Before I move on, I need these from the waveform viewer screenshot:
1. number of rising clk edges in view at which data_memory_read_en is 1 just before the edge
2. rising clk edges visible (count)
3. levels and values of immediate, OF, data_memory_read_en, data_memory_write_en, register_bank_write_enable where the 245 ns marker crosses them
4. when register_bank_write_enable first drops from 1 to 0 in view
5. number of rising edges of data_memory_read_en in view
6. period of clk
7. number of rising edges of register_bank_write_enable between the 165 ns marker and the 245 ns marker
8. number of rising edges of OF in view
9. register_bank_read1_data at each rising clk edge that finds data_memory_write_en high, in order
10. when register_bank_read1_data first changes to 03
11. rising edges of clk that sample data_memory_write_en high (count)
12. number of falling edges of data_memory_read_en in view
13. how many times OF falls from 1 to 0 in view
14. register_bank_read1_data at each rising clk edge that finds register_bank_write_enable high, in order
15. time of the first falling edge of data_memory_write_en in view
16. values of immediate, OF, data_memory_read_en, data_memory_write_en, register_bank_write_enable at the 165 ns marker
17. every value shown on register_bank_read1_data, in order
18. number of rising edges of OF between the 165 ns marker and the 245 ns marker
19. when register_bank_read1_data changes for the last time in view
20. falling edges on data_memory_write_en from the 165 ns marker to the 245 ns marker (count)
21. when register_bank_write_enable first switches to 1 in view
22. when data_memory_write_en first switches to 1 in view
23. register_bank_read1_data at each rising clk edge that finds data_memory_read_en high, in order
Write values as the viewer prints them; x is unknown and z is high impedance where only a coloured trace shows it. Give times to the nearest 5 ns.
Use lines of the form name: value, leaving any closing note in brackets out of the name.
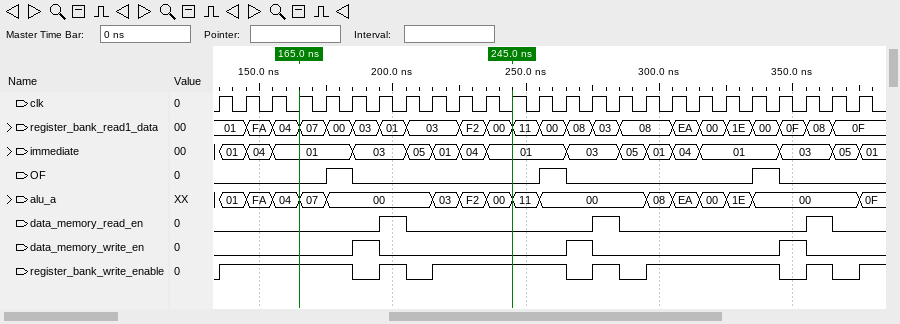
number of rising clk edges in view at which data_memory_read_en is 1 just before the edge: 3
rising clk edges visible: 25
levels and values of immediate, OF, data_memory_read_en, data_memory_write_en, register_bank_write_enable where the 245 ns marker crosses them: immediate=01, OF=0, data_memory_read_en=0, data_memory_write_en=0, register_bank_write_enable=1
when register_bank_write_enable first drops from 1 to 0 in view: 185 ns
number of rising edges of data_memory_read_en in view: 3
period of clk: 10 ns
number of rising edges of register_bank_write_enable between the 165 ns marker and the 245 ns marker: 2
number of rising edges of OF in view: 3
register_bank_read1_data at each rising clk edge that finds data_memory_write_en high, in order: 03, 08, 0F
when register_bank_read1_data first changes to 03: 185 ns
rising edges of clk that sample data_memory_write_en high: 3
number of falling edges of data_memory_read_en in view: 3
how many times OF falls from 1 to 0 in view: 3
register_bank_read1_data at each rising clk edge that finds register_bank_write_enable high, in order: 01, FA, 04, 07, 00, 01, 03, F2, 00, 11, 00, 03, 08, EA, 00, 1E, 00, 08
time of the first falling edge of data_memory_write_en in view: 195 ns
values of immediate, OF, data_memory_read_en, data_memory_write_en, register_bank_write_enable at the 165 ns marker: immediate=01, OF=0, data_memory_read_en=0, data_memory_write_en=0, register_bank_write_enable=1
every value shown on register_bank_read1_data, in order: 01, FA, 04, 07, 00, 03, 01, 03, F2, 00, 11, 00, 08, 03, 08, EA, 00, 1E, 00, 0F, 08, 0F
number of rising edges of OF between the 165 ns marker and the 245 ns marker: 1
when register_bank_read1_data changes for the last time in view: 365 ns
falling edges on data_memory_write_en from the 165 ns marker to the 245 ns marker: 1
when register_bank_write_enable first switches to 1 in view: 135 ns
when data_memory_write_en first switches to 1 in view: 185 ns
register_bank_read1_data at each rising clk edge that finds data_memory_read_en high, in order: 01, 03, 08
